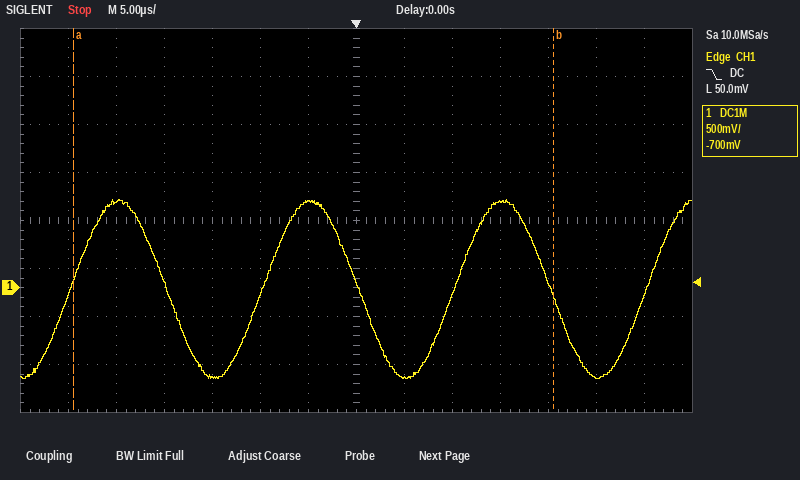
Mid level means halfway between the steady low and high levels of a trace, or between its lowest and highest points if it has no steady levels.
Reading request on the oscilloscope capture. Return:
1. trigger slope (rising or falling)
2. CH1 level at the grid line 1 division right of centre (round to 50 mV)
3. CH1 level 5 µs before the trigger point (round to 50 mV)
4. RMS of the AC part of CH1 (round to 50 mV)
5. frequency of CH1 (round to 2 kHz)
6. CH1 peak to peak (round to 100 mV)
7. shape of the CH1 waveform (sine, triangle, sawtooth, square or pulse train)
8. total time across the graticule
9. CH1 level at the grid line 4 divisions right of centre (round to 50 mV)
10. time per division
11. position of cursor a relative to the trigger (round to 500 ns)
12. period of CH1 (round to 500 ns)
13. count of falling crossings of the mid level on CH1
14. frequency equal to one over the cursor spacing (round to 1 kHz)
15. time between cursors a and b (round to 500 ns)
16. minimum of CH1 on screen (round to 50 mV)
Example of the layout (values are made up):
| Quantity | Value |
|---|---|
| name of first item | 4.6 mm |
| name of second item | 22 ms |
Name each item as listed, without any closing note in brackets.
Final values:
| Quantity | Value |
|---|---|
| trigger slope | falling |
| CH1 level at the grid line 1 division right of centre | -950 mV |
| CH1 level 5 µs before the trigger point | 900 mV |
| RMS of the AC part of CH1 | 650 mV |
| frequency of CH1 | 50 kHz |
| CH1 peak to peak | 1.90 V |
| shape of the CH1 waveform | sine |
| total time across the graticule | 70 µs |
| CH1 level at the grid line 4 divisions right of centre | 50 mV |
| time per division | 5 µs |
| position of cursor a relative to the trigger | -29.5 µs |
| period of CH1 | 20.0 µs |
| count of falling crossings of the mid level on CH1 | 3 |
| frequency equal to one over the cursor spacing | 20 kHz |
| time between cursors a and b | 50.0 µs |
| minimum of CH1 on screen | -950 mV |
